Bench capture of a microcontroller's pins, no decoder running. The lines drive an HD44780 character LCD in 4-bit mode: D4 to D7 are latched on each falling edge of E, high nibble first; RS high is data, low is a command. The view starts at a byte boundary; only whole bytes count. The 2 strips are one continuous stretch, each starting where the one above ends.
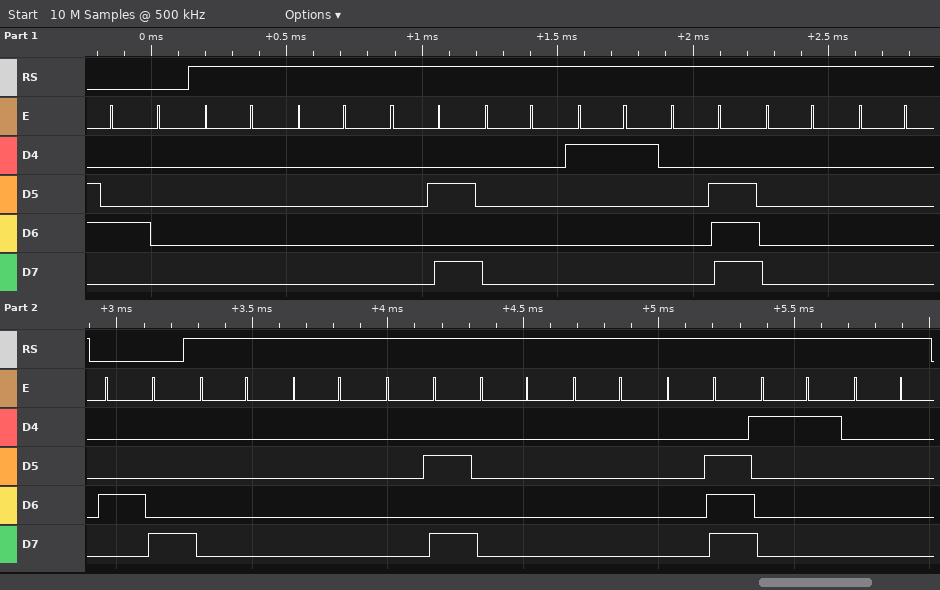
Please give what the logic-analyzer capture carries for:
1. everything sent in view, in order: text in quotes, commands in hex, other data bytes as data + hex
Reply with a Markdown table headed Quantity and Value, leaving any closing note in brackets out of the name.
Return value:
| Quantity | Value |
|---|---|
| everything sent in view, in order: text in quotes, commands in hex, other data bytes as data + hex | 0x40 data 00 00 0A 00 11 0E 00 00 0x48 data 00 00 0A 00 00 0E 11 00 |
